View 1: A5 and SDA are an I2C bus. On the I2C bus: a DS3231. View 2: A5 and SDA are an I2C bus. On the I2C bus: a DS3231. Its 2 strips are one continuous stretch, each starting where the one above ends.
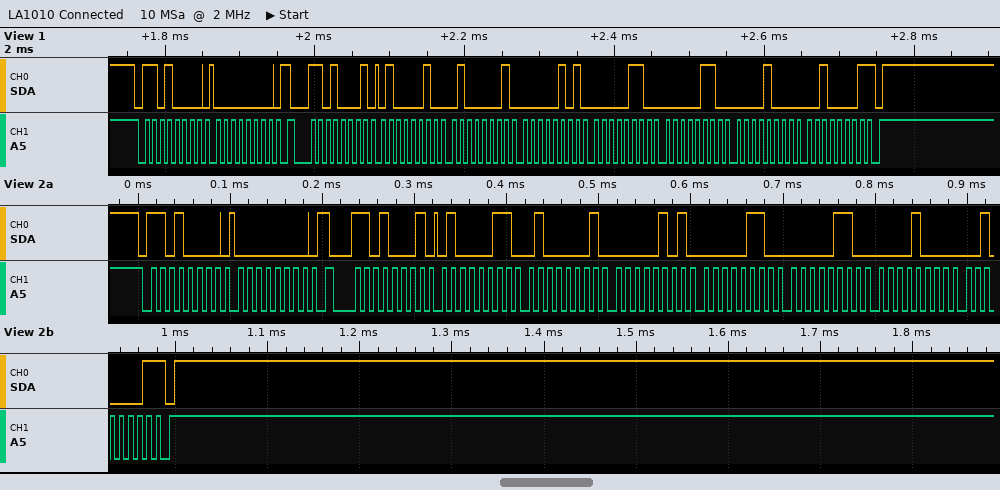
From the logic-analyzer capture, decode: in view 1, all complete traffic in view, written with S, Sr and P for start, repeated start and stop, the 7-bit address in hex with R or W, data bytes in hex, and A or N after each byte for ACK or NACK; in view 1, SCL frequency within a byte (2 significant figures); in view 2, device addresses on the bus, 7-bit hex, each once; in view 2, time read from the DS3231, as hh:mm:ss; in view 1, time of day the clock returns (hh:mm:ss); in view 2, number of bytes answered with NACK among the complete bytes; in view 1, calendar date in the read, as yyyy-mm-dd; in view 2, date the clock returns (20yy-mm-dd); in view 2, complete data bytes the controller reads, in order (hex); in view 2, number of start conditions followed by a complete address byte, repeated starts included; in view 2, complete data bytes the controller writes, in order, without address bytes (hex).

S 68W A 00 A Sr 68R A 42 A 41 A 05 A 06 A 06 A 08 A 21 N P
100 kHz
0x68
05:41:43
05:41:42
1
2021-08-06
2021-08-06
43 41 05 06 06 08 21
2
00
